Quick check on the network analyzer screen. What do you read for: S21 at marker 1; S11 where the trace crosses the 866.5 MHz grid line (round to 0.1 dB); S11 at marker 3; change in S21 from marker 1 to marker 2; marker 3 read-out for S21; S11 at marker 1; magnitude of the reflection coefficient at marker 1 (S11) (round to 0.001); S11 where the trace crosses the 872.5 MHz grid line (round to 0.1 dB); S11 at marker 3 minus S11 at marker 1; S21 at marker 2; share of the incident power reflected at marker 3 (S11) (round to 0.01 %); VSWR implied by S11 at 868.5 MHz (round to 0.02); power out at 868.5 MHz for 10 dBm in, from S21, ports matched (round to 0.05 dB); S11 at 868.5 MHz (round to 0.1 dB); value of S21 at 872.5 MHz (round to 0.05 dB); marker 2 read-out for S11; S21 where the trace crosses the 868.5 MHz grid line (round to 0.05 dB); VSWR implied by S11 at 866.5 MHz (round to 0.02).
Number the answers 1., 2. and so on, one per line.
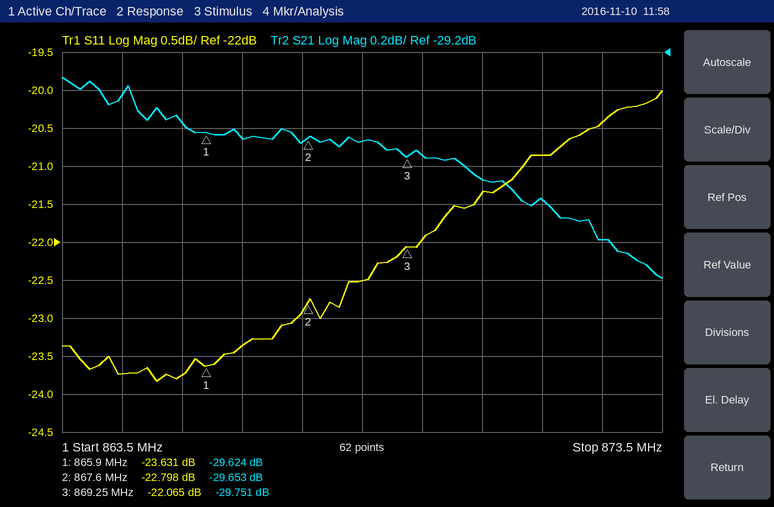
1. -29.624 dB
2. -23.4 dB
3. -22.065 dB
4. -0.029 dB
5. -29.751 dB
6. -23.631 dB
7. 0.066
8. -20.4 dB
9. 1.566 dB
10. -29.653 dB
11. 0.62 %
12. 1.16
13. -19.65 dBm
14. -22.5 dB
15. -30.20 dB
16. -22.798 dB
17. -29.65 dB
18. 1.14
